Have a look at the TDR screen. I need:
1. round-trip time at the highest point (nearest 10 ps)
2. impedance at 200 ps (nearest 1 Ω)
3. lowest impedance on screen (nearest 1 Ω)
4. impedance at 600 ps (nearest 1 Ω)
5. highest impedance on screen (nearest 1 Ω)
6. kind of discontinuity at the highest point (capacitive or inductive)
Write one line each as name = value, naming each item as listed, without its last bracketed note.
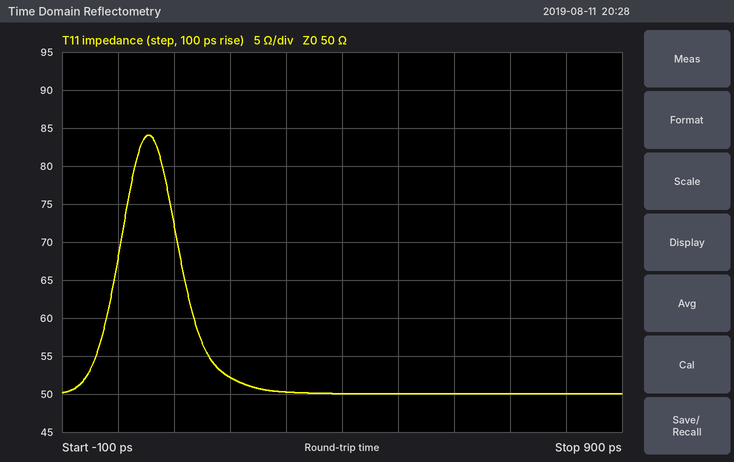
round-trip time at the highest point = 50 ps
impedance at 200 ps = 52 Ω
lowest impedance on screen = 50 Ω
impedance at 600 ps = 50 Ω
highest impedance on screen = 84 Ω
kind of discontinuity at the highest point = inductive
